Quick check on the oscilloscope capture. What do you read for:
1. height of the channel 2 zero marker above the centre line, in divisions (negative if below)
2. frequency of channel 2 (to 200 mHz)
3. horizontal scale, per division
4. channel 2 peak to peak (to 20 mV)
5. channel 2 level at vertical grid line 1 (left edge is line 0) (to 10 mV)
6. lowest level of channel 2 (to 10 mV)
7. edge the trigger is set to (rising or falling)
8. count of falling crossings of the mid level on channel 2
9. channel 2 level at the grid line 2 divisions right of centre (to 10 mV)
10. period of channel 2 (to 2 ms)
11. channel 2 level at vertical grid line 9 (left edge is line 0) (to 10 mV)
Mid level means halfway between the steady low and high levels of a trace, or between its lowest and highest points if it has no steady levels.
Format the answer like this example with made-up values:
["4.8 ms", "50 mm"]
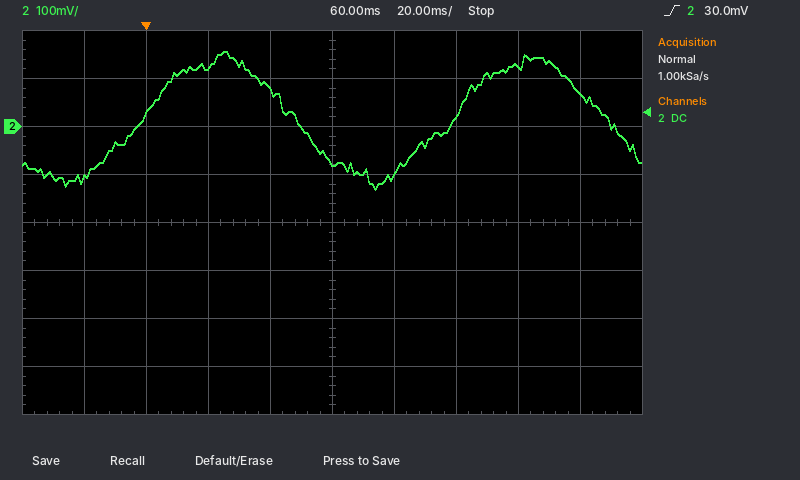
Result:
["+2.0 div", "10.0 Hz", "20 ms", "280 mV", "-110 mV", "-130 mV", "rising", "2", "20 mV", "100 ms", "70 mV"]
